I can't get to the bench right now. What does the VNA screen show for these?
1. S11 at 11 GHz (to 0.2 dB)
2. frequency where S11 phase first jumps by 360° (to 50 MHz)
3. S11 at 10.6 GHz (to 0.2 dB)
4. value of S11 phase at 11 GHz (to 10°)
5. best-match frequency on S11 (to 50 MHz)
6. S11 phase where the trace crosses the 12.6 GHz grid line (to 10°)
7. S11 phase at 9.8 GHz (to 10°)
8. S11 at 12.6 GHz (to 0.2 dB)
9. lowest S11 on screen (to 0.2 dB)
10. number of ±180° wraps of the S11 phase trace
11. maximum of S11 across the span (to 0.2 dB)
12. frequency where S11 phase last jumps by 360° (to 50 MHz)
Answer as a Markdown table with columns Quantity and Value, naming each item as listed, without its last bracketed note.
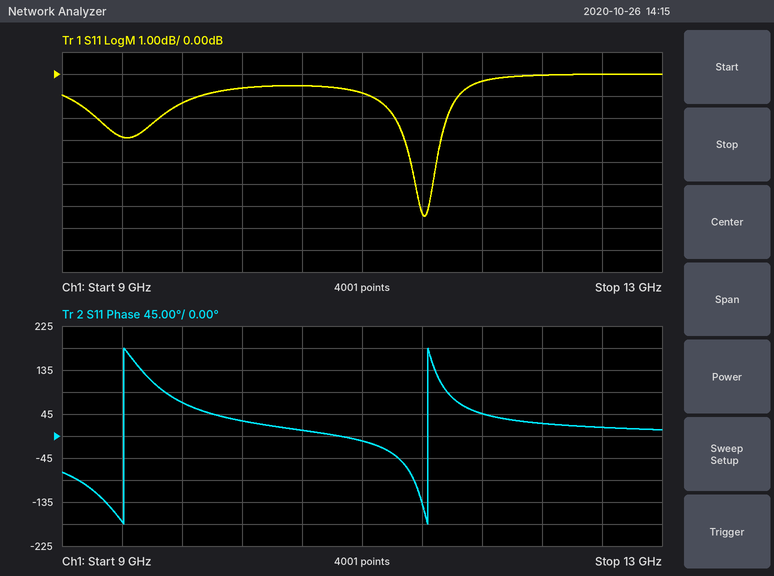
| Quantity | Value |
|---|---|
| S11 at 11 GHz | -0.8 dB |
| frequency where S11 phase first jumps by 360° | 9.40 GHz |
| S11 at 10.6 GHz | -0.6 dB |
| value of S11 phase at 11 GHz | -10° |
| best-match frequency on S11 | 11.40 GHz |
| S11 phase where the trace crosses the 12.6 GHz grid line | 20° |
| S11 phase at 9.8 GHz | 70° |
| S11 at 12.6 GHz | 0.0 dB |
| lowest S11 on screen | -6.4 dB |
| number of ±180° wraps of the S11 phase trace | 2 |
| maximum of S11 across the span | 0.0 dB |
| frequency where S11 phase last jumps by 360° | 11.45 GHz |
